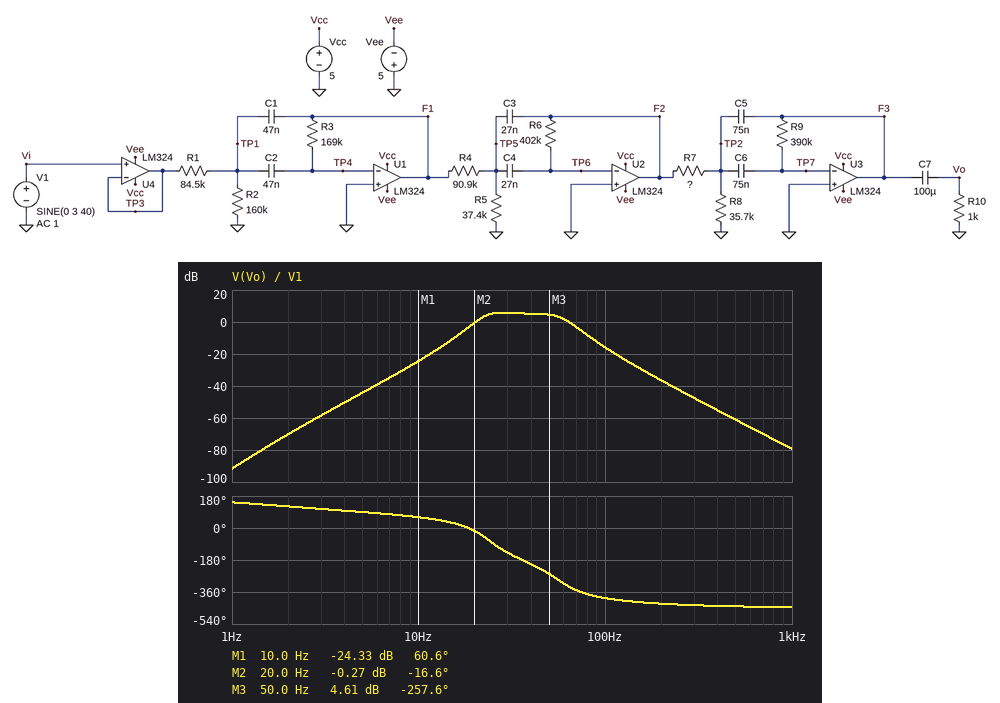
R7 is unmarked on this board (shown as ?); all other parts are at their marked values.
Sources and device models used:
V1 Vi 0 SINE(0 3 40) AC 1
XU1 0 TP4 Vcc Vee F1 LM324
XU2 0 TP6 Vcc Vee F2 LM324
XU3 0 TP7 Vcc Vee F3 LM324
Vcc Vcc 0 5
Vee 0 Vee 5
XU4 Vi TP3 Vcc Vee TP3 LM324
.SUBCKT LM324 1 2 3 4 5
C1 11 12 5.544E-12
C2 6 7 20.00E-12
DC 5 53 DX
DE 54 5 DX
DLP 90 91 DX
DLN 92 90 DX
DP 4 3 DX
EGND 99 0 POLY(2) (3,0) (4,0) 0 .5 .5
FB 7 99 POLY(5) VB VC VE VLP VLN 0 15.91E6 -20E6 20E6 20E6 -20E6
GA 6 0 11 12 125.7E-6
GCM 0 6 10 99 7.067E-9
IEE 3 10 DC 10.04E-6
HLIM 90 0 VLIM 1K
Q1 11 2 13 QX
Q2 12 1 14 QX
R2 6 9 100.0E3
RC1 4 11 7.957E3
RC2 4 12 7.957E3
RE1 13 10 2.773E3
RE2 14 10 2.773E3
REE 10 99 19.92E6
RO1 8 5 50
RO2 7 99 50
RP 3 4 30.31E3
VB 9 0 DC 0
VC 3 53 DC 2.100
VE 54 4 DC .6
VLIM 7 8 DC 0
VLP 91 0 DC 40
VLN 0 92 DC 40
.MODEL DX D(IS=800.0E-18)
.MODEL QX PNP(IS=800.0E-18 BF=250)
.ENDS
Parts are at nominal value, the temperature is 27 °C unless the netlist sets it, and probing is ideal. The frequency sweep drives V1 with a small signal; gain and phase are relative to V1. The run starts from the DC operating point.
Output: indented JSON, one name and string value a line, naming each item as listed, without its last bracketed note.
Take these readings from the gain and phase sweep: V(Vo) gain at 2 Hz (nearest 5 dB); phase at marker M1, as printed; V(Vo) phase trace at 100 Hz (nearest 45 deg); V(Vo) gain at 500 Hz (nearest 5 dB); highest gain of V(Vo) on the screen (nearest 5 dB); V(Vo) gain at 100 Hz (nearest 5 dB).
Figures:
{
  "V(Vo) gain at 2 Hz": "-70 dB",
  "phase at marker M1, as printed": "60.6 deg",
  "V(Vo) phase trace at 100 Hz": "-405 deg",
  "V(Vo) gain at 500 Hz": "-60 dB",
  "highest gain of V(Vo) on the screen": "5 dB",
  "V(Vo) gain at 100 Hz": "-15 dB"
}
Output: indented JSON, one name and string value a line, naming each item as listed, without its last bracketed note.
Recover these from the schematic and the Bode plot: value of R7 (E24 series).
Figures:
{
  "value of R7": "51 kΩ"
}
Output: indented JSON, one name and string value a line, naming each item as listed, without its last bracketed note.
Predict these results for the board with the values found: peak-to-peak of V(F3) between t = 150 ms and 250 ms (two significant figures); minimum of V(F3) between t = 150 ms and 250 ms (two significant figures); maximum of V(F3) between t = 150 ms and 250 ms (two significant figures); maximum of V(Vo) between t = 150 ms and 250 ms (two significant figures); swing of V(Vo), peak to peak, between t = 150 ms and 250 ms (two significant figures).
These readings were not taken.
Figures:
{
  "peak-to-peak of V(F3) between t = 150 ms and 250 ms": "8.3 V",
  "minimum of V(F3) between t = 150 ms and 250 ms": "-4.8 V",
  "maximum of V(F3) between t = 150 ms and 250 ms": "3.5 V",
  "maximum of V(Vo) between t = 150 ms and 250 ms": "3.8 V",
  "swing of V(Vo), peak to peak, between t = 150 ms and 250 ms": "8.4 V"
}
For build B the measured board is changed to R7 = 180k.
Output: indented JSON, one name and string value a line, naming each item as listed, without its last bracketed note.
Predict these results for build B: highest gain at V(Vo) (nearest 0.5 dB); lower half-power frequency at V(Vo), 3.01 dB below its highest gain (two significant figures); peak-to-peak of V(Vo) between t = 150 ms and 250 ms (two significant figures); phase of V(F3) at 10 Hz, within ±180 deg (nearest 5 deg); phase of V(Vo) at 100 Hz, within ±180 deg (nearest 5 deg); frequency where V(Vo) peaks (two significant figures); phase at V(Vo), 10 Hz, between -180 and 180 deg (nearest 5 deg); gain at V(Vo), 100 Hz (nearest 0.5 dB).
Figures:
{
  "highest gain at V(Vo)": "-7.0 dB",
  "lower half-power frequency at V(Vo), 3.01 dB below its highest gain": "20 Hz",
  "peak-to-peak of V(Vo) between t = 150 ms and 250 ms": "2.7 V",
  "phase of V(F3) at 10 Hz, within ±180 deg": "45 deg",
  "phase of V(Vo) at 100 Hz, within ±180 deg": "-35 deg",
  "frequency where V(Vo) peaks": "45 Hz",
  "phase at V(Vo), 10 Hz, between -180 and 180 deg": "55 deg",
  "gain at V(Vo), 100 Hz": "-27.0 dB"
}
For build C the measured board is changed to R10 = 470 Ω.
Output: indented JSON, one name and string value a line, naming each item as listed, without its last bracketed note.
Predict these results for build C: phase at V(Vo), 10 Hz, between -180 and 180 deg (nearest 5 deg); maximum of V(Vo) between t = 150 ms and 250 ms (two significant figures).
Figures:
{
  "phase at V(Vo), 10 Hz, between -180 and 180 deg": "70 deg",
  "maximum of V(Vo) between t = 150 ms and 250 ms": "3.9 V"
}
